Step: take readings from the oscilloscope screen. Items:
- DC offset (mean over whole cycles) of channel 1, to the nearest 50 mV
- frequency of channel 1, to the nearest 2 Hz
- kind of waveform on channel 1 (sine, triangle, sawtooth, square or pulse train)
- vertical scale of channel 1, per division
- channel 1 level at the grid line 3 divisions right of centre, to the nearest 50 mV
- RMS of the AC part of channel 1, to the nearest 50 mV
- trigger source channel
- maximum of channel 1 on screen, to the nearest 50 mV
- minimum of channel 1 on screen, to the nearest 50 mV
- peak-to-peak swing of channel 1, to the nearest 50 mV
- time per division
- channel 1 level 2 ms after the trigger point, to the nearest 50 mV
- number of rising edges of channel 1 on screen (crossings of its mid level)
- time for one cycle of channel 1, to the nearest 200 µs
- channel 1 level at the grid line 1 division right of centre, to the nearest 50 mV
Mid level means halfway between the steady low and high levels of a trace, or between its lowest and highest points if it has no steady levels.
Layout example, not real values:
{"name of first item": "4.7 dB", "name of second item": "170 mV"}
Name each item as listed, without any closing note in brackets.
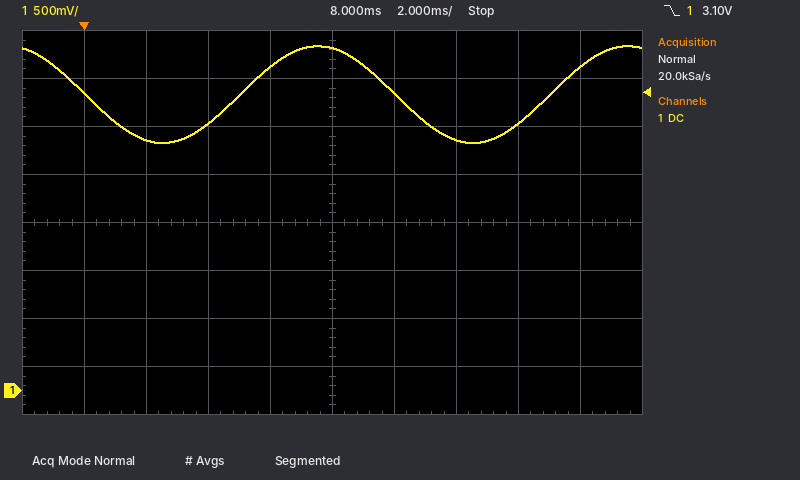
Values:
{"DC offset (mean over whole cycles) of channel 1, to the nearest 50 mV": "3.10 V", "frequency of channel 1, to the nearest 2 Hz": "100 Hz", "kind of waveform on channel 1": "sine", "vertical scale of channel 1, per division": "500 mV", "channel 1 level at the grid line 3 divisions right of centre, to the nearest 50 mV": "2.80 V", "RMS of the AC part of channel 1, to the nearest 50 mV": "350 mV", "trigger source channel": "channel 1", "maximum of channel 1 on screen, to the nearest 50 mV": "3.60 V", "minimum of channel 1 on screen, to the nearest 50 mV": "2.60 V", "peak-to-peak swing of channel 1, to the nearest 50 mV": "1.00 V", "time per division": "2 ms", "channel 1 level 2 ms after the trigger point, to the nearest 50 mV": "2.60 V", "number of rising edges of channel 1 on screen": "2", "time for one cycle of channel 1, to the nearest 200 µs": "10.0 ms", "channel 1 level at the grid line 1 division right of centre, to the nearest 50 mV": "3.10 V"}
